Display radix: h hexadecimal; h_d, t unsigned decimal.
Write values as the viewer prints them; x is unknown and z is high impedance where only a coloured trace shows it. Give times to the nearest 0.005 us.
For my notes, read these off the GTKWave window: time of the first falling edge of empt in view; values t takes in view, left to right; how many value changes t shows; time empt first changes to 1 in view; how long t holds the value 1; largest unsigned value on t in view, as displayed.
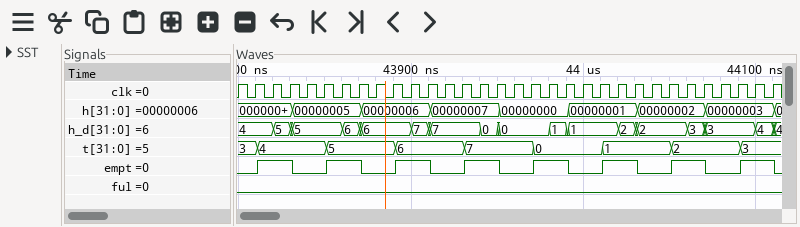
43.83 us
3, 4, 5, 6, 7, 0, 1, 2, 3
8
43.81 us
0.04 us
7
